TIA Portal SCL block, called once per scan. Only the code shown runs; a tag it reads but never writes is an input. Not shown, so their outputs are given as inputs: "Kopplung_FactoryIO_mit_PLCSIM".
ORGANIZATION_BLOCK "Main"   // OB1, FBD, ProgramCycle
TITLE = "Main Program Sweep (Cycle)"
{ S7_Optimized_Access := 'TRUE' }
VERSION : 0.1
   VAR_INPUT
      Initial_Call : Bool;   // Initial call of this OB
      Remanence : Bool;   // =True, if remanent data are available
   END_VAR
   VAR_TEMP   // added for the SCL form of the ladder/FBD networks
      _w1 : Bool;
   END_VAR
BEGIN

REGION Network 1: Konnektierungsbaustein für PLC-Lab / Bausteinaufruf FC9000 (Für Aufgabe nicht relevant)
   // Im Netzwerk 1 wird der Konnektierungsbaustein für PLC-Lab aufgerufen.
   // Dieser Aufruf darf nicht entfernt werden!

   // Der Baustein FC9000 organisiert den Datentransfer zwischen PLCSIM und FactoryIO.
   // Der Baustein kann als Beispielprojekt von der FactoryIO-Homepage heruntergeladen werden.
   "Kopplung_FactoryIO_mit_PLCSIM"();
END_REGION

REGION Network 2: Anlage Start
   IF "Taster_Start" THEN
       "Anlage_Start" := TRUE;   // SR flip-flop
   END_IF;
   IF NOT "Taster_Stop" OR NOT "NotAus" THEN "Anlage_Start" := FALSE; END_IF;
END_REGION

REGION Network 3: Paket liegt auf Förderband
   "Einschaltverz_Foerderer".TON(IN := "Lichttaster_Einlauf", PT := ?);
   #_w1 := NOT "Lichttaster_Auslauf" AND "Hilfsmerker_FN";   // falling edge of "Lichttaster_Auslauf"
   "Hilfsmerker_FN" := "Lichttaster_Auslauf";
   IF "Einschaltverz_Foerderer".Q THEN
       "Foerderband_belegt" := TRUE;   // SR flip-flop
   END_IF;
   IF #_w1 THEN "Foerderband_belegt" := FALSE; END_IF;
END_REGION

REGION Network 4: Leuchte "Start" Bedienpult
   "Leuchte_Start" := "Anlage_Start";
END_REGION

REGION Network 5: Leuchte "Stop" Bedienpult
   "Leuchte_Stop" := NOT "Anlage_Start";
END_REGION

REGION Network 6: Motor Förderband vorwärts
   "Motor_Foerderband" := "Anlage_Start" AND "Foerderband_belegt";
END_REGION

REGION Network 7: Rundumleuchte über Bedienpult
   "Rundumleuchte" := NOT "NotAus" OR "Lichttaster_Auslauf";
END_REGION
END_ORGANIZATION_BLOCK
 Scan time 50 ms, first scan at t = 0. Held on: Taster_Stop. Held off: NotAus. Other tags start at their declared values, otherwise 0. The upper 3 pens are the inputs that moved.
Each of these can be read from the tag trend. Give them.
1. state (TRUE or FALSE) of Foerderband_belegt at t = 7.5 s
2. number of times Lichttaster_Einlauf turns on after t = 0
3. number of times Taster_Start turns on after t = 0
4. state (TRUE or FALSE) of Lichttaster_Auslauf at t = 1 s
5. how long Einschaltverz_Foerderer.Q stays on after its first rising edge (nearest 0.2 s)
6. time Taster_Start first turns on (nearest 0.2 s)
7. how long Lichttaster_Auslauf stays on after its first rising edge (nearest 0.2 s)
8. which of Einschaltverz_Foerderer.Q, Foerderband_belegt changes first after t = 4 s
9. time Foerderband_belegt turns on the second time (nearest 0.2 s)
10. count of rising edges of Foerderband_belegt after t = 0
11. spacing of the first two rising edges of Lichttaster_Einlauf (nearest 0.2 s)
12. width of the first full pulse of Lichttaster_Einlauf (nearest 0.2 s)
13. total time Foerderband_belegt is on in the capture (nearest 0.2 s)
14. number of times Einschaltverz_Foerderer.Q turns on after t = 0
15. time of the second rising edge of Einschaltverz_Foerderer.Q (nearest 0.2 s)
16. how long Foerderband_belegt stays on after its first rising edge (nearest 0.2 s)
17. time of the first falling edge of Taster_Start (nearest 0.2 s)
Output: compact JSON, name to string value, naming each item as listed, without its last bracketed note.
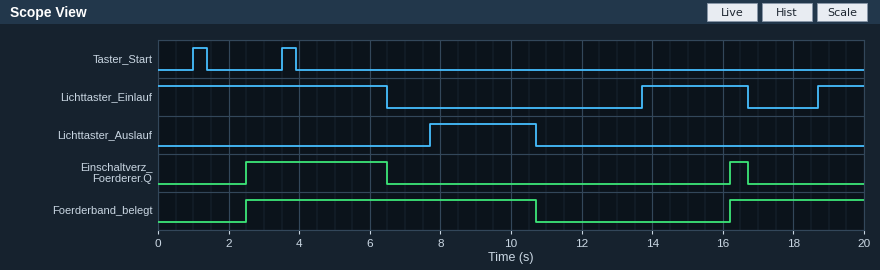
{"state (TRUE or FALSE) of Foerderband_belegt at t = 7.5 s": "TRUE", "number of times Lichttaster_Einlauf turns on after t = 0": "2", "number of times Taster_Start turns on after t = 0": "2", "state (TRUE or FALSE) of Lichttaster_Auslauf at t = 1 s": "FALSE", "how long Einschaltverz_Foerderer.Q stays on after its first rising edge": "4.0 s", "time Taster_Start first turns on": "1.0 s", "how long Lichttaster_Auslauf stays on after its first rising edge": "3.0 s", "which of Einschaltverz_Foerderer.Q, Foerderband_belegt changes first after t = 4 s": "Einschaltverz_Foerderer.Q", "time Foerderband_belegt turns on the second time": "16.2 s", "count of rising edges of Foerderband_belegt after t = 0": "2", "spacing of the first two rising edges of Lichttaster_Einlauf": "5.0 s", "width of the first full pulse of Lichttaster_Einlauf": "3.0 s", "total time Foerderband_belegt is on in the capture": "12.0 s", "number of times Einschaltverz_Foerderer.Q turns on after t = 0": "2", "time of the second rising edge of Einschaltverz_Foerderer.Q": "16.2 s", "how long Foerderband_belegt stays on after its first rising edge": "8.2 s", "time of the first falling edge of Taster_Start": "1.4 s"}
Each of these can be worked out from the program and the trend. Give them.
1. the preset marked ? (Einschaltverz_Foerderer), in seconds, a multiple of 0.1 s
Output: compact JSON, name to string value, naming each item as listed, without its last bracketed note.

{"the preset marked ? (Einschaltverz_Foerderer), in seconds, a multiple of 0.1 s": "2.5 s"}
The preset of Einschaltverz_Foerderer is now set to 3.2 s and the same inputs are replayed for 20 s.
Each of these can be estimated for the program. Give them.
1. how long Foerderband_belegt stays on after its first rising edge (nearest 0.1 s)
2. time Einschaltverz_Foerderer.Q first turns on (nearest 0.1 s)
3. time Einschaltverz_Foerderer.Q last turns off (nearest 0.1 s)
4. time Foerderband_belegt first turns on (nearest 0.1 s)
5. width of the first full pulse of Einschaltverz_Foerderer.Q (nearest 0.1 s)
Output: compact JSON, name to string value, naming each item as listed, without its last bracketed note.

{"how long Foerderband_belegt stays on after its first rising edge": "7.5 s", "time Einschaltverz_Foerderer.Q first turns on": "3.2 s", "time Einschaltverz_Foerderer.Q last turns off": "6.5 s", "time Foerderband_belegt first turns on": "3.2 s", "width of the first full pulse of Einschaltverz_Foerderer.Q": "3.3 s"}
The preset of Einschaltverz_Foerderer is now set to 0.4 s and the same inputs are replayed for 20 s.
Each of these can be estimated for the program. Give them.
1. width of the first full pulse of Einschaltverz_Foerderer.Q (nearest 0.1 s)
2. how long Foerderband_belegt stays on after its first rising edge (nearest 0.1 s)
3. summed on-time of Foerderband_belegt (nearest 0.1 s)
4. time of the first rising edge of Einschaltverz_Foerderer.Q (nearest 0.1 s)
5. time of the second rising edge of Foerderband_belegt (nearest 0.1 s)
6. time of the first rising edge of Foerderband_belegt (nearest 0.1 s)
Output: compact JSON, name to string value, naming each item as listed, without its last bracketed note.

{"width of the first full pulse of Einschaltverz_Foerderer.Q": "6.1 s", "how long Foerderband_belegt stays on after its first rising edge": "10.3 s", "summed on-time of Foerderband_belegt": "16.2 s", "time of the first rising edge of Einschaltverz_Foerderer.Q": "0.4 s", "time of the second rising edge of Foerderband_belegt": "14.1 s", "time of the first rising edge of Foerderband_belegt": "0.4 s"}
